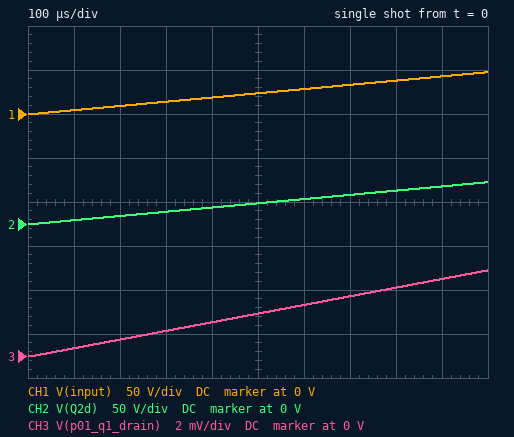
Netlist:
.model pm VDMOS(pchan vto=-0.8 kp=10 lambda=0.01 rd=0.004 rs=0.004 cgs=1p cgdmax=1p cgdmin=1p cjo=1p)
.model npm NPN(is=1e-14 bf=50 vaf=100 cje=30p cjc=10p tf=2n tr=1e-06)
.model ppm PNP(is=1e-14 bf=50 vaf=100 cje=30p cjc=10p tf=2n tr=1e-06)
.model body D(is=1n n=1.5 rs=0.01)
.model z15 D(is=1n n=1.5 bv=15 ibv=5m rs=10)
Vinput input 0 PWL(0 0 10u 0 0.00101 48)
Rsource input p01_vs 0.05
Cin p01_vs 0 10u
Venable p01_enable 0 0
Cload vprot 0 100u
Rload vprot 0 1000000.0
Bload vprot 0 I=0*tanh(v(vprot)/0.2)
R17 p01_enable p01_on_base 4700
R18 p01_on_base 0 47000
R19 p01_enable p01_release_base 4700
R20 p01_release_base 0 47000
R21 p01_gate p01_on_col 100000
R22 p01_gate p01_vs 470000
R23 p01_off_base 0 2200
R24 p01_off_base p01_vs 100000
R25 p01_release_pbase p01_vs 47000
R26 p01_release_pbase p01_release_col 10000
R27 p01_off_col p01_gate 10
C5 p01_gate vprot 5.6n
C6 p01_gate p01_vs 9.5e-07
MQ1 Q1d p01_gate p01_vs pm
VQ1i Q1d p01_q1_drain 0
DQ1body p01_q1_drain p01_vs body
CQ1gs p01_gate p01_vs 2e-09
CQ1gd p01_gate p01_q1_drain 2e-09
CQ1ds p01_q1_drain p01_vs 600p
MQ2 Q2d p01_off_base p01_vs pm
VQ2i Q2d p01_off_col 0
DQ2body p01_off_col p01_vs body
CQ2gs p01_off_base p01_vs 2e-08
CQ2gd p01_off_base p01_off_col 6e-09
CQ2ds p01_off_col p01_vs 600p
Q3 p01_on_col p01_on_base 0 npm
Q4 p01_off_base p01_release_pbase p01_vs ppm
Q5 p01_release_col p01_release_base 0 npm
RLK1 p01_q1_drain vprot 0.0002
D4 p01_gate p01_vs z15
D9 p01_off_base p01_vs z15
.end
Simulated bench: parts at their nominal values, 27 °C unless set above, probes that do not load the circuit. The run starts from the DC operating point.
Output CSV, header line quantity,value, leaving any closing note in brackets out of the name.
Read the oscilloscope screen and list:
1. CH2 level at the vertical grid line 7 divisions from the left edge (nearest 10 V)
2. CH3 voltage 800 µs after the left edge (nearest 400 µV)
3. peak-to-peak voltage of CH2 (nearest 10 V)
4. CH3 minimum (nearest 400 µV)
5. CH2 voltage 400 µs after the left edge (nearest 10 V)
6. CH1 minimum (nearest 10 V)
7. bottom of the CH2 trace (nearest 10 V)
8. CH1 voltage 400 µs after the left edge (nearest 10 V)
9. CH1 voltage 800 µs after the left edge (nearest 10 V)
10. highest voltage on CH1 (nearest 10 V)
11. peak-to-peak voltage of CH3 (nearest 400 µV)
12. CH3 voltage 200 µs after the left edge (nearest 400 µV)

quantity,value
CH2 level at the vertical grid line 7 divisions from the left edge,30 V
CH3 voltage 800 µs after the left edge,3.2 mV
peak-to-peak voltage of CH2,50 V
CH3 minimum,0 V
CH2 voltage 400 µs after the left edge,20 V
CH1 minimum,0 V
bottom of the CH2 trace,0 V
CH1 voltage 400 µs after the left edge,20 V
CH1 voltage 800 µs after the left edge,40 V
highest voltage on CH1,50 V
peak-to-peak voltage of CH3,4.0 mV
CH3 voltage 200 µs after the left edge,800 µV
